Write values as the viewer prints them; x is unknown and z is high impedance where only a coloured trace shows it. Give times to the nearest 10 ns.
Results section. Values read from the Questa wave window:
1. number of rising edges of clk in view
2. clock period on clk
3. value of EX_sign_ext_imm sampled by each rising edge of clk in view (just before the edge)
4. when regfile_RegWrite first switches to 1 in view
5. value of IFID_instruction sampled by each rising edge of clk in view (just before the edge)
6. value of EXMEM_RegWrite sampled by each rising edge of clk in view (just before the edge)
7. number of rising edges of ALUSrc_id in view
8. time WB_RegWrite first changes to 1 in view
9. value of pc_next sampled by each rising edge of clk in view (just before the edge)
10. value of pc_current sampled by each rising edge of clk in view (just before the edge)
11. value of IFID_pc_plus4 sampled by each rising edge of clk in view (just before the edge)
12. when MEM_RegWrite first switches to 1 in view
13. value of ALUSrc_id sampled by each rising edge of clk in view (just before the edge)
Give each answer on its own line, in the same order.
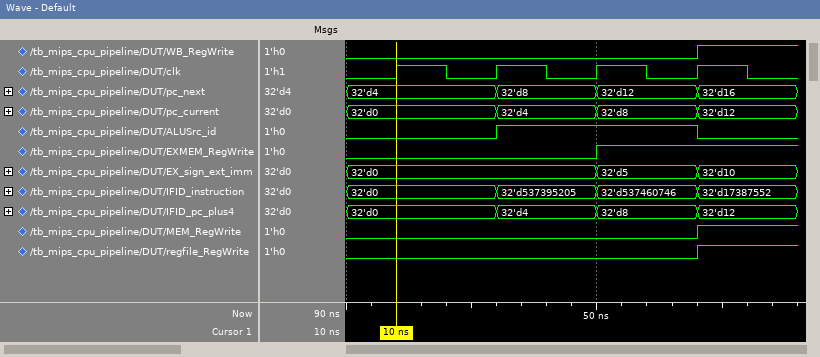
4
20 ns
32'd0, 32'd0, 32'd0, 32'd5
70 ns
32'd0, 32'd0, 32'd537395205, 32'd537460746
0 0 0 1
1
70 ns
32'd4, 32'd4, 32'd8, 32'd12
32'd0, 32'd0, 32'd4, 32'd8
32'd0, 32'd0, 32'd4, 32'd8
70 ns
0 0 1 1
